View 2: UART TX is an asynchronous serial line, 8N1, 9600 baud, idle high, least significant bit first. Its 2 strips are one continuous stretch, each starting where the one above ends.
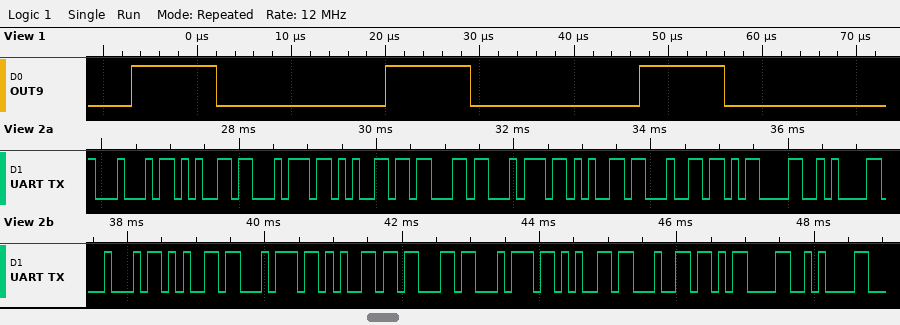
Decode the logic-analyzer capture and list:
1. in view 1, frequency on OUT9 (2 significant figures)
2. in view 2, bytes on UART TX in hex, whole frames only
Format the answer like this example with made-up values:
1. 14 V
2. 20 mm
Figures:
1. 37 kHz
2. 44 65 74 65 63 74 65 64 0D 0A 44 65 74 65 63 74 65 64 0D 0A
